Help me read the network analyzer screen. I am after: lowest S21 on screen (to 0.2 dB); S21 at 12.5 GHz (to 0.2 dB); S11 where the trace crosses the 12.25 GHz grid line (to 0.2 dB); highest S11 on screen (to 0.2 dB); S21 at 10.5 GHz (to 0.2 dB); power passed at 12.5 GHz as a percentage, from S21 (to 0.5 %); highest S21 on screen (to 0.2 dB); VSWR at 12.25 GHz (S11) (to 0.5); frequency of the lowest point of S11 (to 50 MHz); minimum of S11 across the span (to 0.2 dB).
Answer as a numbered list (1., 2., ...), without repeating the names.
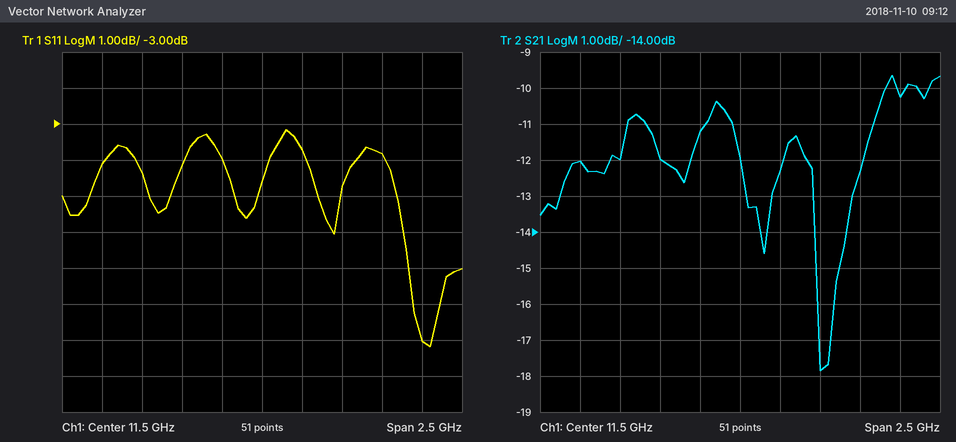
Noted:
1. -17.8 dB
2. -10.2 dB
3. -3.8 dB
4. -3.2 dB
5. -12.0 dB
6. 9.5 %
7. -9.6 dB
8. 4.5
9. 12.55 GHz
10. -9.2 dB
